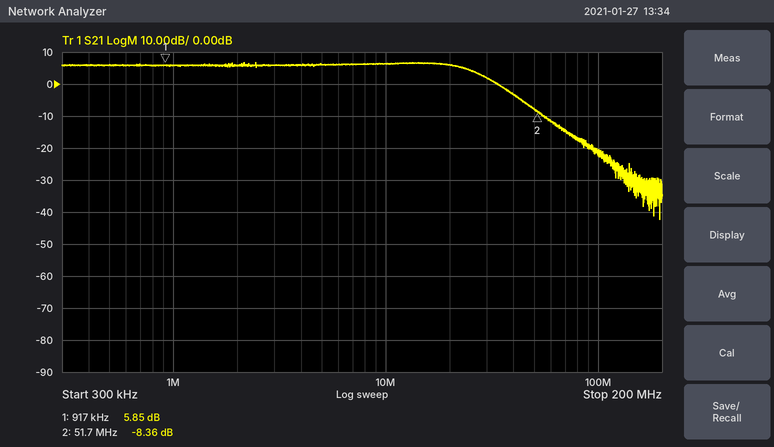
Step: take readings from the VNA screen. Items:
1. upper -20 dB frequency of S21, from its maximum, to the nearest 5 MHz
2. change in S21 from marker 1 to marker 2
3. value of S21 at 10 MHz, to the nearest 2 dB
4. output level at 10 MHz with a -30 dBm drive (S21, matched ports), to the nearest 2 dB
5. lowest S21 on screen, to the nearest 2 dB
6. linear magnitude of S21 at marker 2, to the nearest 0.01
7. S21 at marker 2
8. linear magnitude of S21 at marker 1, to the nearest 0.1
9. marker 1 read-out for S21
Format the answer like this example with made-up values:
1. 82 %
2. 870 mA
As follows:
1. 65 MHz
2. -14.21 dB
3. 6 dB
4. -24 dBm
5. -42 dB
6. 0.38
7. -8.36 dB
8. 2.0
9. 5.85 dB
